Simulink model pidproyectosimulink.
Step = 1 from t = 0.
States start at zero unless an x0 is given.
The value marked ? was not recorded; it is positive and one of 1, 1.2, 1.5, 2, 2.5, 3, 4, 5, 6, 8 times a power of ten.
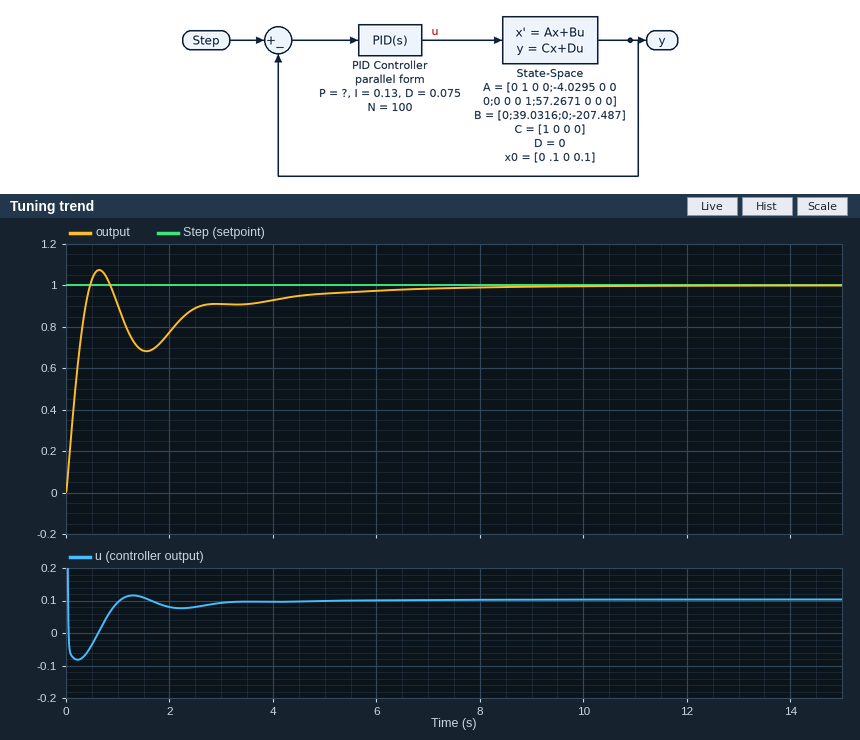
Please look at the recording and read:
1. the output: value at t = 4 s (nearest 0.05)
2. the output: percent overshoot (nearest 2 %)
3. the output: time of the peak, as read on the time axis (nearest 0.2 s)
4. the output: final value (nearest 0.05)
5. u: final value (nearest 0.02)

0.95
8 %
0.6 s
1.00
0.10
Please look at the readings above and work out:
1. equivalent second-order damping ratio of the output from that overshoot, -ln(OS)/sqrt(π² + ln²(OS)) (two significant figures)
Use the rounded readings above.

0.63
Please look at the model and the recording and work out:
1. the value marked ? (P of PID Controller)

0.2
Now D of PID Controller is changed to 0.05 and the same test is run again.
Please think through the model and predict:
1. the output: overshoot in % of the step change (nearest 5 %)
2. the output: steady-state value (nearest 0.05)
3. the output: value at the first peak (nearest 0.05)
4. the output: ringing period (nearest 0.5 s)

15 %
1.00
1.15
2.0 s
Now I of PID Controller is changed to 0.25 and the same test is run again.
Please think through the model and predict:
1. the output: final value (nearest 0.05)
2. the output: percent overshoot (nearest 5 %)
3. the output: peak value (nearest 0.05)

1.00
15 %
1.15
